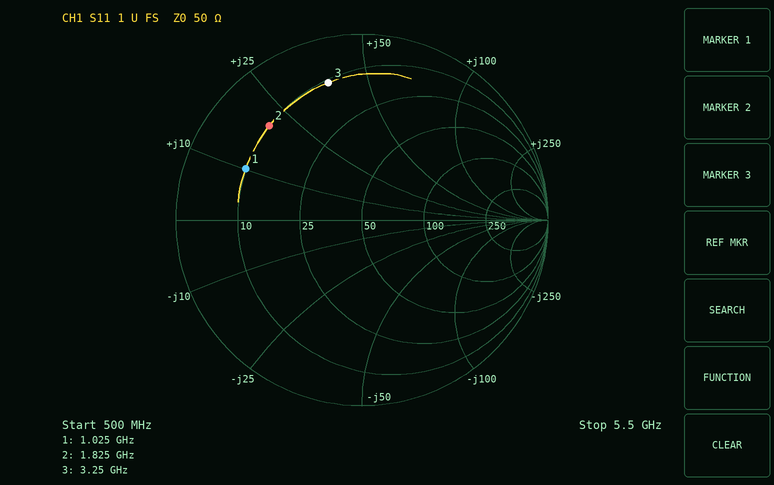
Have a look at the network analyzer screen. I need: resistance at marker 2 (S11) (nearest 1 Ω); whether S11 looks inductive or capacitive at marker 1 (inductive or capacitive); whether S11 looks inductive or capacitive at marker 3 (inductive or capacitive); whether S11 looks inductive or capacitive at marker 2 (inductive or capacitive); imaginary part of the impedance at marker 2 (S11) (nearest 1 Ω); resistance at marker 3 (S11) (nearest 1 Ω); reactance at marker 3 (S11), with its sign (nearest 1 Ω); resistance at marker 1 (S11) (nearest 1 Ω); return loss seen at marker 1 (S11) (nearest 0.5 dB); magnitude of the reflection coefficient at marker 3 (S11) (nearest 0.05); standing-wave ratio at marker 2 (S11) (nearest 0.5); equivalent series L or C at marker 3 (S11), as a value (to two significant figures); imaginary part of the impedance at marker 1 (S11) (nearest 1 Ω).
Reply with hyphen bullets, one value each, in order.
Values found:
- 10 Ω
- inductive
- inductive
- inductive
- +20 Ω
- 11 Ω
- +38 Ω
- 10 Ω
- 3.5 dB
- 0.75
- 6.0
- 1.9 nH
- +10 Ω
